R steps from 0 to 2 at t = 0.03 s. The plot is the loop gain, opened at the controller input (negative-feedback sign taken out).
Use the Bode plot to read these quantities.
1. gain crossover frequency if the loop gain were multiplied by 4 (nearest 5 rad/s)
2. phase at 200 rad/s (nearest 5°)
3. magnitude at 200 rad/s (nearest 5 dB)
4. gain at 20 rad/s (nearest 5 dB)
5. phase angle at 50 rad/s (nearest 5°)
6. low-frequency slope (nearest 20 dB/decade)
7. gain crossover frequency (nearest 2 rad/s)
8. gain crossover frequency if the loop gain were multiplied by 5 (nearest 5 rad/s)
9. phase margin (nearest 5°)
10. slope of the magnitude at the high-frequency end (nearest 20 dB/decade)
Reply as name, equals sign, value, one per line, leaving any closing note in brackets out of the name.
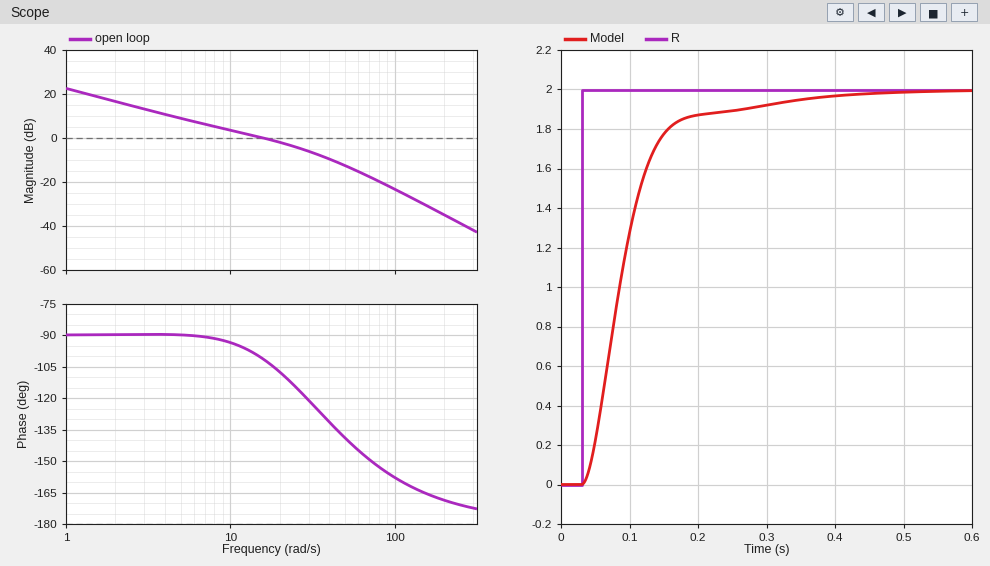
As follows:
gain crossover frequency if the loop gain were multiplied by 4 = 50 rad/s
phase at 200 rad/s = -170°
magnitude at 200 rad/s = -35 dB
gain at 20 rad/s = 0 dB
phase angle at 50 rad/s = -140°
low-frequency slope = -20 dB/decade
gain crossover frequency = 16 rad/s
gain crossover frequency if the loop gain were multiplied by 5 = 55 rad/s
phase margin = 80°
slope of the magnitude at the high-frequency end = -40 dB/decade
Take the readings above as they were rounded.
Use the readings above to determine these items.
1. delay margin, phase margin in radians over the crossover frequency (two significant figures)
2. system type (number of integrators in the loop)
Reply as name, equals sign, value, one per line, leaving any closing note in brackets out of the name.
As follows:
delay margin, phase margin in radians over the crossover frequency = 0.087 s
system type = 1
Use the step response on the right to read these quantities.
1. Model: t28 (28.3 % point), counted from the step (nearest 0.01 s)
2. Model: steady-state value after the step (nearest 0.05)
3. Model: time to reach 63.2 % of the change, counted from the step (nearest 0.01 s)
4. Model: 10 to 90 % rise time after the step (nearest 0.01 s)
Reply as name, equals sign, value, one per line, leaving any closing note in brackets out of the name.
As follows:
Model: t28 (28.3 % point), counted from the step = 0.04 s
Model: steady-state value after the step = 2.00
Model: time to reach 63.2 % of the change, counted from the step = 0.07 s
Model: 10 to 90 % rise time after the step = 0.11 s
